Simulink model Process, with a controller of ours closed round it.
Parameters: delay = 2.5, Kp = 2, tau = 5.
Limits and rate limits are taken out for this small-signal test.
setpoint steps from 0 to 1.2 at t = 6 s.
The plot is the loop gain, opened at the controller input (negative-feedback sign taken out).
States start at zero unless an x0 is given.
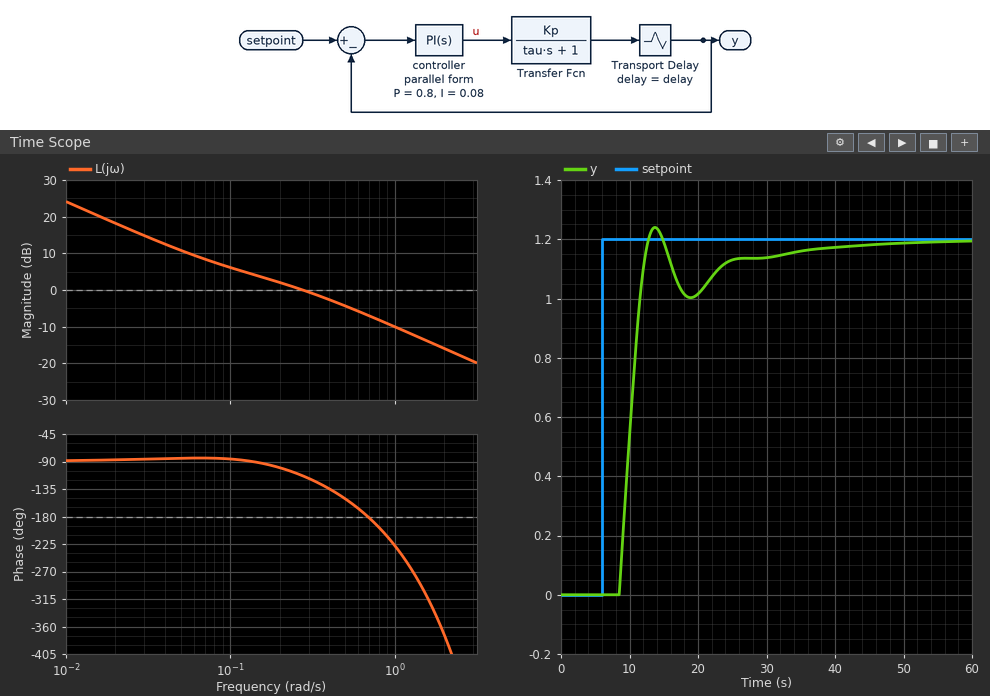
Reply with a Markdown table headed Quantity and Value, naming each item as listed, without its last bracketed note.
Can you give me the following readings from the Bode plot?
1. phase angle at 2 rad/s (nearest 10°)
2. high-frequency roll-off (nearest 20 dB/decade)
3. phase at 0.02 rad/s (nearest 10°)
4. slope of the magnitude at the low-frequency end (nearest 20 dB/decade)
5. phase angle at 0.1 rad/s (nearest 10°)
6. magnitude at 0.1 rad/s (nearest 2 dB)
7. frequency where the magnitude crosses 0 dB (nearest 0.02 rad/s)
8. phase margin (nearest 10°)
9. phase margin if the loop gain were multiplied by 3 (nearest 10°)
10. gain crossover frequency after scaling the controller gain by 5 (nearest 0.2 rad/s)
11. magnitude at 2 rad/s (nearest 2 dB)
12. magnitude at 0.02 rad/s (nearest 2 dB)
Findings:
| Quantity | Value |
|---|---|
| phase angle at 2 rad/s | -370° |
| high-frequency roll-off | -20 dB/decade |
| phase at 0.02 rad/s | -90° |
| slope of the magnitude at the low-frequency end | -20 dB/decade |
| phase angle at 0.1 rad/s | -90° |
| magnitude at 0.1 rad/s | 6 dB |
| frequency where the magnitude crosses 0 dB | 0.28 rad/s |
| phase margin | 70° |
| phase margin if the loop gain were multiplied by 3 | -40° |
| gain crossover frequency after scaling the controller gain by 5 | 1.6 rad/s |
| magnitude at 2 rad/s | -16 dB |
| magnitude at 0.02 rad/s | 18 dB |
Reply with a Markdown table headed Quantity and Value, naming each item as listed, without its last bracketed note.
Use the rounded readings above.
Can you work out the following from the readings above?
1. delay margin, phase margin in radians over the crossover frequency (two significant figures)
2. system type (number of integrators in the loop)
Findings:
| Quantity | Value |
|---|---|
| delay margin, phase margin in radians over the crossover frequency | 4.4 s |
| system type | 1 |
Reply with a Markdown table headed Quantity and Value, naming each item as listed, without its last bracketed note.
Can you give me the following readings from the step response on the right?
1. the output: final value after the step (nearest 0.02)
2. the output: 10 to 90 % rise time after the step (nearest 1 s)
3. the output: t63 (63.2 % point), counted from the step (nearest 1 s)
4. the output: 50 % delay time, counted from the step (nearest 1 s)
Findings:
| Quantity | Value |
|---|---|
| the output: final value after the step | 1.20 |
| the output: 10 to 90 % rise time after the step | 3 s |
| the output: t63 (63.2 % point), counted from the step | 5 s |
| the output: 50 % delay time, counted from the step | 4 s |
